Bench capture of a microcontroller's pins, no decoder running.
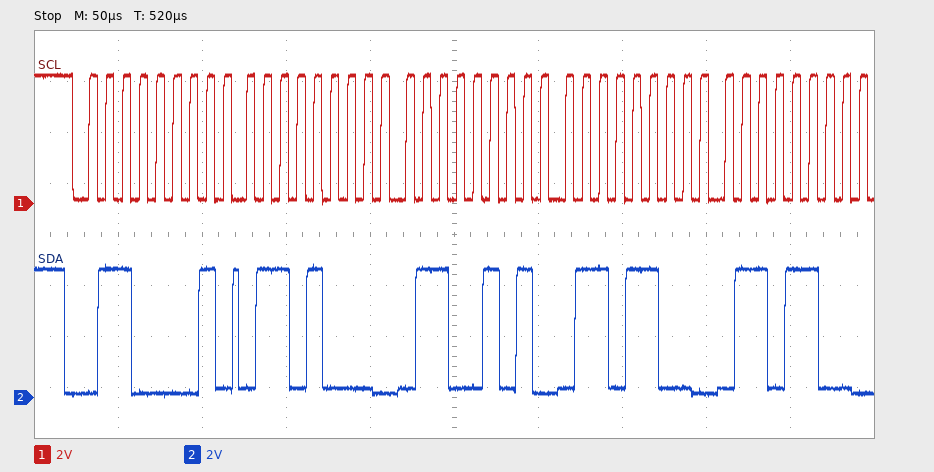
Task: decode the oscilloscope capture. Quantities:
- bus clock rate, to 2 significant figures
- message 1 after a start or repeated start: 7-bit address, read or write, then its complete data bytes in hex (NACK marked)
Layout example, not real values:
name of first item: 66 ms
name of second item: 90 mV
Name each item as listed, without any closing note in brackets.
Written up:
bus clock rate, to 2 significant figures: 100 kHz
message 1 after a start or repeated start: 7-bit address, read or write, then its complete data bytes in hex: 0x30 read: 68 65 6C 6C
